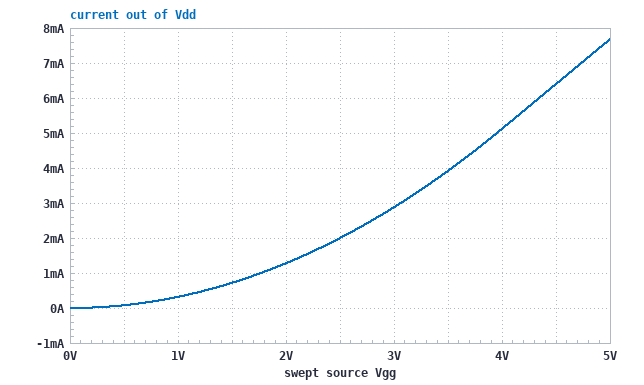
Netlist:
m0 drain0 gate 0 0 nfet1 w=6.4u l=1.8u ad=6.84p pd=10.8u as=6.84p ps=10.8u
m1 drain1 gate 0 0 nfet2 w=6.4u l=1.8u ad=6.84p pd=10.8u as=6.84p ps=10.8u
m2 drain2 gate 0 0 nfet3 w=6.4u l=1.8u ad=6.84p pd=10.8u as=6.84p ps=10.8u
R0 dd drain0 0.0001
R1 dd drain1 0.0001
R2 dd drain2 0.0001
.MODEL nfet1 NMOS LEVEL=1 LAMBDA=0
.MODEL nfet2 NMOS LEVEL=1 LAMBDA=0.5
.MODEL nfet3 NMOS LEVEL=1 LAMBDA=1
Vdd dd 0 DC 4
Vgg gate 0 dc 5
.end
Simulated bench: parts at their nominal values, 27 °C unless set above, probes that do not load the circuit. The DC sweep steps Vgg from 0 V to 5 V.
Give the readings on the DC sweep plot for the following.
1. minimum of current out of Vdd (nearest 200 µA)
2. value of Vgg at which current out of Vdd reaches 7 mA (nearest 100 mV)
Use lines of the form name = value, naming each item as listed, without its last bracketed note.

minimum of current out of Vdd = 0 A
value of Vgg at which current out of Vdd reaches 7 mA = 4.7 V
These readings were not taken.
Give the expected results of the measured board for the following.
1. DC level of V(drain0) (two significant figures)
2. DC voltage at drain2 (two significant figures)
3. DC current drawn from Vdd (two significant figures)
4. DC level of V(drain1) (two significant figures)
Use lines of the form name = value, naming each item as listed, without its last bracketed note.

DC level of V(drain0) = 4.0 V
DC voltage at drain2 = 4.0 V
DC current drawn from Vdd = 7.7 mA
DC level of V(drain1) = 4.0 V
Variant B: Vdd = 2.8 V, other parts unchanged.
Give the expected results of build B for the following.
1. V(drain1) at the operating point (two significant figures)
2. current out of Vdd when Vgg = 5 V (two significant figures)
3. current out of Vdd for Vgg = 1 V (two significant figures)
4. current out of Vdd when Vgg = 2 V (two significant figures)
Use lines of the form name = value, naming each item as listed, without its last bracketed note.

V(drain1) at the operating point = 2.8 V
current out of Vdd when Vgg = 5 V = 5.2 mA
current out of Vdd for Vgg = 1 V = 260 µA
current out of Vdd when Vgg = 2 V = 1.0 mA
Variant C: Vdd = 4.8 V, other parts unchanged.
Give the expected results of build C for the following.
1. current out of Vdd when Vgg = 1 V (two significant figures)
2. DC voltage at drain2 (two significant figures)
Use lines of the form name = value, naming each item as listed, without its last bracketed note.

current out of Vdd when Vgg = 1 V = 360 µA
DC voltage at drain2 = 4.8 V
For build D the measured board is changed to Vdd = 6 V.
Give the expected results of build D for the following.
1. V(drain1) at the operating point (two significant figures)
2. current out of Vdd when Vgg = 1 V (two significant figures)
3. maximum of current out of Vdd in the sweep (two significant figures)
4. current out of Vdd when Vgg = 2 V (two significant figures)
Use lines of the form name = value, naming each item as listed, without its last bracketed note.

V(drain1) at the operating point = 6.0 V
current out of Vdd when Vgg = 1 V = 430 µA
maximum of current out of Vdd in the sweep = 11 mA
current out of Vdd when Vgg = 2 V = 1.7 mA
